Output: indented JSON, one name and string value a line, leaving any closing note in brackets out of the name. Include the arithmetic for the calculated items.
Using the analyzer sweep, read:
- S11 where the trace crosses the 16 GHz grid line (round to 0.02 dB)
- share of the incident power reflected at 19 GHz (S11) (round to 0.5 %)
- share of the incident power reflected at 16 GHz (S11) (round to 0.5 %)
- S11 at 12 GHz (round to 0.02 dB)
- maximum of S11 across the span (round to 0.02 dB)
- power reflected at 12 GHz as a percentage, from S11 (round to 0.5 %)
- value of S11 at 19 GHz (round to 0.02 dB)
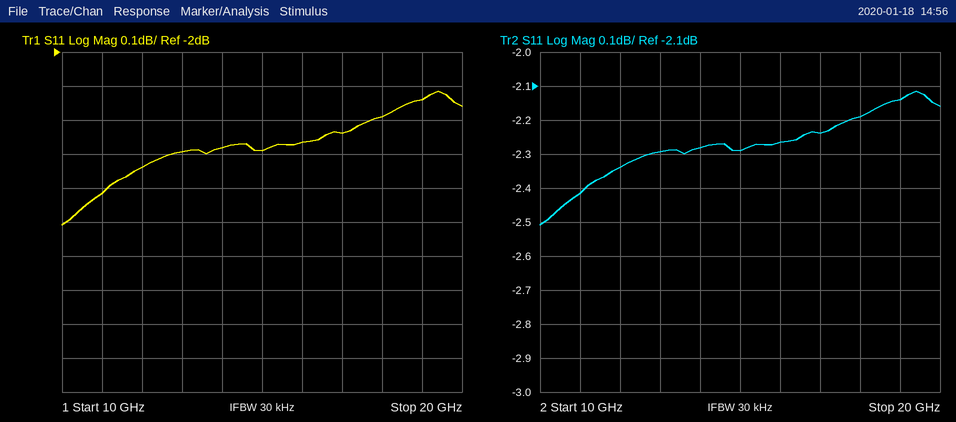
{
  "S11 where the trace crosses the 16 GHz grid line": "-2.26 dB",
  "share of the incident power reflected at 19 GHz (S11)": "10^(-2.14/10) ≈ 61.1 %, so 61.0 % to the nearest 0.5 %",
  "share of the incident power reflected at 16 GHz (S11)": "10^(-2.26/10) ≈ 59.4 %, so 59.5 % to the nearest 0.5 %",
  "S11 at 12 GHz": "-2.34 dB",
  "maximum of S11 across the span": "-2.12 dB",
  "power reflected at 12 GHz as a percentage, from S11": "10^(-2.34/10) ≈ 58.3 %, so 58.5 % to the nearest 0.5 %",
  "value of S11 at 19 GHz": "-2.14 dB"
}
